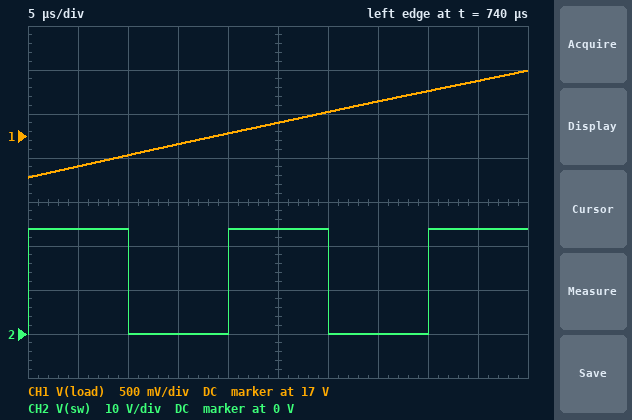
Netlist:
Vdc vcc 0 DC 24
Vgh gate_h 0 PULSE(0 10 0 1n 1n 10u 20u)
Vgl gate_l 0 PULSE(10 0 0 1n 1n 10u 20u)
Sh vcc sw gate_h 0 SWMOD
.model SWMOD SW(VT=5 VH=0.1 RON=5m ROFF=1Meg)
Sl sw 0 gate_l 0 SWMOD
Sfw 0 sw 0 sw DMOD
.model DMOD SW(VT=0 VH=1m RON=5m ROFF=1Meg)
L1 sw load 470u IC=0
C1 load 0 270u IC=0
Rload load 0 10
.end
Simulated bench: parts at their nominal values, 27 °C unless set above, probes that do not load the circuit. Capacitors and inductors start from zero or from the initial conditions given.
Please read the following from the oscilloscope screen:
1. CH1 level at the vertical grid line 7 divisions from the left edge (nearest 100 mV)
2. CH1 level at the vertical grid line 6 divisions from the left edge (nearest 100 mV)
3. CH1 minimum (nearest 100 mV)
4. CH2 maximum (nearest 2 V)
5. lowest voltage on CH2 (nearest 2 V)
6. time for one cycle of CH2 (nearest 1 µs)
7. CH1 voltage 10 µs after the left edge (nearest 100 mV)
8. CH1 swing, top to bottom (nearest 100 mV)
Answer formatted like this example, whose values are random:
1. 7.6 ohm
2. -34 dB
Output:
1. 17.4 V
2. 17.3 V
3. 16.5 V
4. 24 V
5. 0 V
6. 20 µs
7. 16.8 V
8. 1.2 V
